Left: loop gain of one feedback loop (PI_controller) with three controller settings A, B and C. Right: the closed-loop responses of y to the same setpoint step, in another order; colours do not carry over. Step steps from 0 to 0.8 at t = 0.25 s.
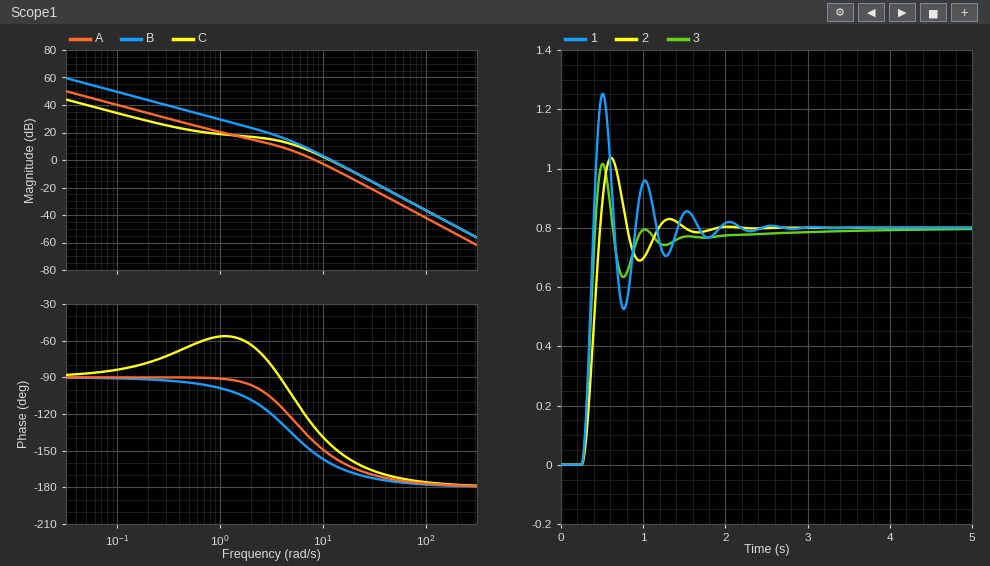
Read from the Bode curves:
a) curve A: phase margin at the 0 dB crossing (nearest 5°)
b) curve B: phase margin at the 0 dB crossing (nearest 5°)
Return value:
35°
20°
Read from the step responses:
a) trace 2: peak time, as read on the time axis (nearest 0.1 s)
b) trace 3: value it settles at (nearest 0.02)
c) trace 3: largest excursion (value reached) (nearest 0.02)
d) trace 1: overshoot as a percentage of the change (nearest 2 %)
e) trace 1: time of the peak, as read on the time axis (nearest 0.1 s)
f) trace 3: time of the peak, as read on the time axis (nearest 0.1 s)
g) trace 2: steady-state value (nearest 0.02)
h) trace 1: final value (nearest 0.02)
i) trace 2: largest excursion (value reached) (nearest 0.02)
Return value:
0.6 s
0.80
1.02
56 %
0.5 s
0.5 s
0.80
0.80
1.04
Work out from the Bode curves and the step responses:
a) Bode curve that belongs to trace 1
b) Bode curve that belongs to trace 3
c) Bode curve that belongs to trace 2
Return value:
B
C
A
